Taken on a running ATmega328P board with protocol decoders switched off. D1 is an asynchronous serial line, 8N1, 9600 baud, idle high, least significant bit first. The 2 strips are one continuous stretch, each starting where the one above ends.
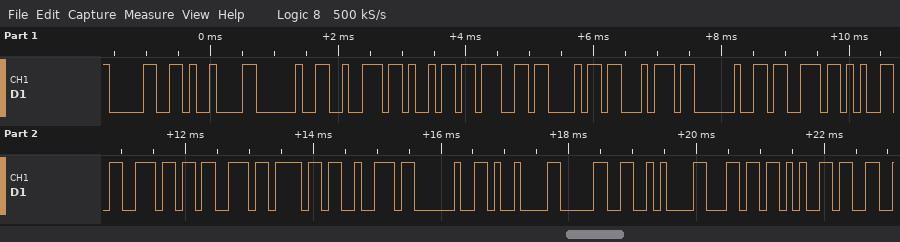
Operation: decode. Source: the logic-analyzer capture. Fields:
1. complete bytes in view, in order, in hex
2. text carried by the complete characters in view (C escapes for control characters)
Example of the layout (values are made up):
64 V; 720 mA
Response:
30 09 20 72 69 67 68 74 20 73 65 6E 73 6F 72 20 09 30 0A 6C 65; "0\t right sensor \t0\nle"
